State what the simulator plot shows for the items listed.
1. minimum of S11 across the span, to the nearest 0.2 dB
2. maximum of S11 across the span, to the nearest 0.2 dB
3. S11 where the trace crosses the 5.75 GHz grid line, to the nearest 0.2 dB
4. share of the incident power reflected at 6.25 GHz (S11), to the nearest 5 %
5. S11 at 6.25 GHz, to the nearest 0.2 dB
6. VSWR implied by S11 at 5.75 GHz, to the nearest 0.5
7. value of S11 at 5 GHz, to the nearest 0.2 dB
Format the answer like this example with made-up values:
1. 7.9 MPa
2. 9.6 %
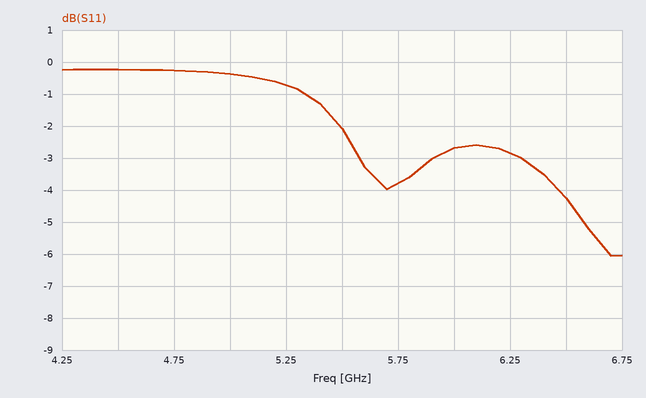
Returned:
1. -6.0 dB
2. -0.2 dB
3. -3.8 dB
4. 50 %
5. -2.8 dB
6. 4.5
7. -0.4 dB
